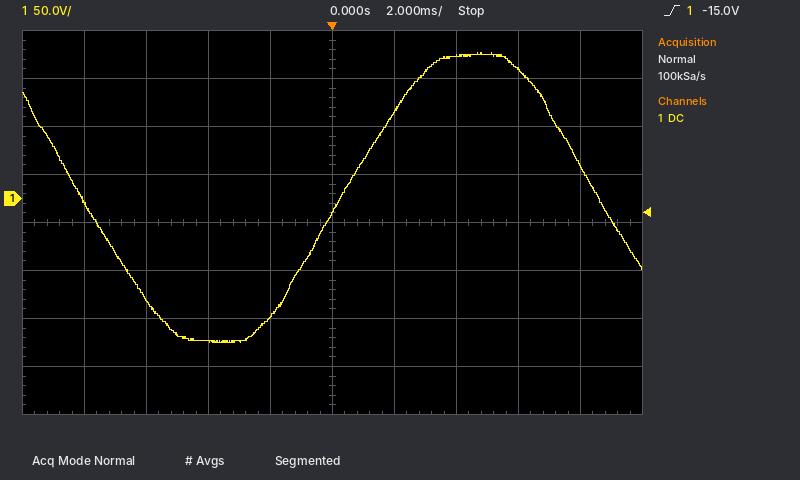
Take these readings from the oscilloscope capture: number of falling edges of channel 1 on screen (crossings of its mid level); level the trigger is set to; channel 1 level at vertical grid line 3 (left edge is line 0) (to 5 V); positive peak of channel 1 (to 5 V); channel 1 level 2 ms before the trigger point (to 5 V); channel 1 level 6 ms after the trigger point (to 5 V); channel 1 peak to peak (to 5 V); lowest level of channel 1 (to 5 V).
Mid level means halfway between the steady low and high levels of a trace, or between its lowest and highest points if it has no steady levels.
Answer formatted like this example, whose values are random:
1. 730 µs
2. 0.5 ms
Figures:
1. 2
2. -15.0 V
3. -150 V
4. 150 V
5. -125 V
6. 135 V
7. 300 V
8. -150 V
